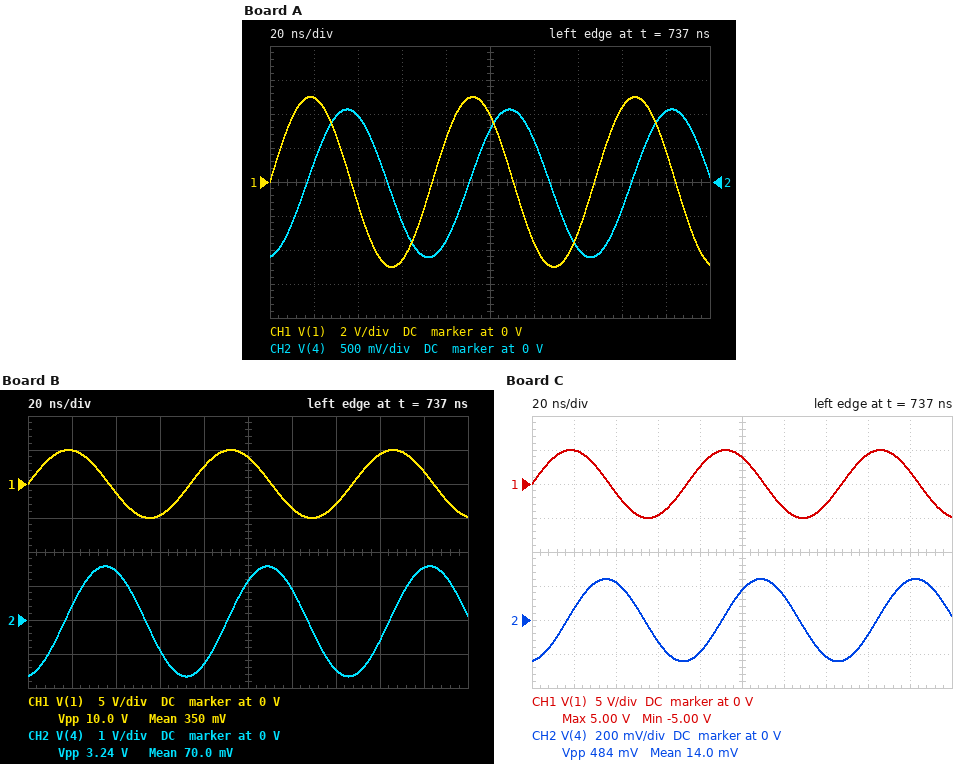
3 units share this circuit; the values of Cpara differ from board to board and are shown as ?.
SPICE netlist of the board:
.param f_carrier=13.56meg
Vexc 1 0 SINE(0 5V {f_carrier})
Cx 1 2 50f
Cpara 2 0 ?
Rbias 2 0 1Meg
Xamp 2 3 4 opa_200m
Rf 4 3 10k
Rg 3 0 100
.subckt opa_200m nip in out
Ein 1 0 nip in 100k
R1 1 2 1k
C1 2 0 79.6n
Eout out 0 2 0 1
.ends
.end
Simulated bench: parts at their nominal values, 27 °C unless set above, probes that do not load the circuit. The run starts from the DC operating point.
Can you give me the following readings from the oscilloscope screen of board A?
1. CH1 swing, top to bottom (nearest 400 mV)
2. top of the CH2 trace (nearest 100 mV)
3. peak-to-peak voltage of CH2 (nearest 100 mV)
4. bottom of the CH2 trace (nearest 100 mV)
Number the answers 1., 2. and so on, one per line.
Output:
1. 10.0 V
2. 1.1 V
3. 2.2 V
4. -1.1 V
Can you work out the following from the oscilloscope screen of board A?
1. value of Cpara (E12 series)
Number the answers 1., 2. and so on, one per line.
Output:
1. 3.3 pF
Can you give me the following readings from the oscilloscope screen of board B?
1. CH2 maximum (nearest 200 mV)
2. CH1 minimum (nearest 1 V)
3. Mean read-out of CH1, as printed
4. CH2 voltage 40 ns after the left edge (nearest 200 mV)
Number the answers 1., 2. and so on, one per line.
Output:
1. 1.6 V
2. -5 V
3. 350 mV
4. 1.4 V
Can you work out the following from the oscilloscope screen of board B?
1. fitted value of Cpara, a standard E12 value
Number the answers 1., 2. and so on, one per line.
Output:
1. 2.2 pF
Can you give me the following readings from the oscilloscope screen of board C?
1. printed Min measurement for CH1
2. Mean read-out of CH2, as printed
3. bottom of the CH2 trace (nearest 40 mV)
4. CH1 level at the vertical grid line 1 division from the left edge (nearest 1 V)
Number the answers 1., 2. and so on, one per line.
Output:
1. -5.00 V
2. 14.0 mV
3. -240 mV
4. 5 V
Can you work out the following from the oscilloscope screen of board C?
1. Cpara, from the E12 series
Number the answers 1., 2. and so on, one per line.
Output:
1. 15 pF
